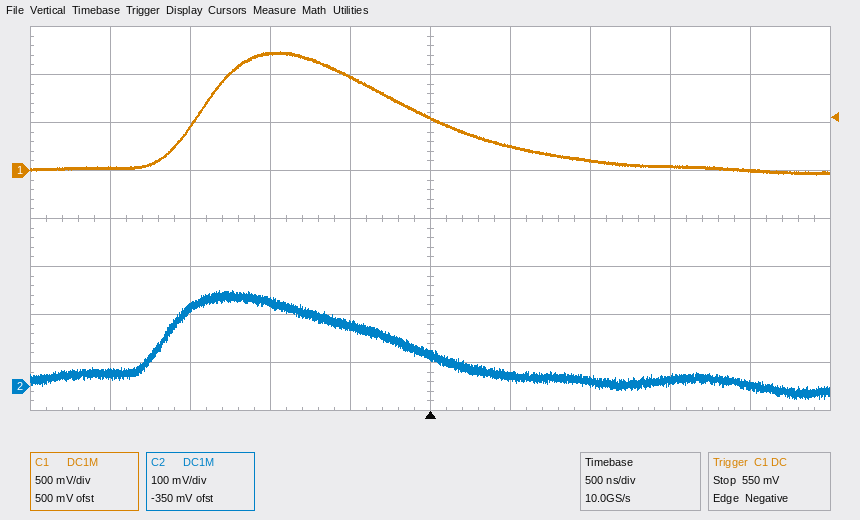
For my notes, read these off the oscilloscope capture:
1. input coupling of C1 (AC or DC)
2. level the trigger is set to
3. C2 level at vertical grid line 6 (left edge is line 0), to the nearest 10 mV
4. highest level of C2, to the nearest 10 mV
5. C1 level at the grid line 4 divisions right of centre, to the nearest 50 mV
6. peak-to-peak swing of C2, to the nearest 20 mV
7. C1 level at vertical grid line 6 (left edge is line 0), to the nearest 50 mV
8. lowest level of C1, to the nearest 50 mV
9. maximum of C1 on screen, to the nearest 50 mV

DC
550 mV
20 mV
200 mV
0 mV
220 mV
250 mV
-50 mV
1.25 V
